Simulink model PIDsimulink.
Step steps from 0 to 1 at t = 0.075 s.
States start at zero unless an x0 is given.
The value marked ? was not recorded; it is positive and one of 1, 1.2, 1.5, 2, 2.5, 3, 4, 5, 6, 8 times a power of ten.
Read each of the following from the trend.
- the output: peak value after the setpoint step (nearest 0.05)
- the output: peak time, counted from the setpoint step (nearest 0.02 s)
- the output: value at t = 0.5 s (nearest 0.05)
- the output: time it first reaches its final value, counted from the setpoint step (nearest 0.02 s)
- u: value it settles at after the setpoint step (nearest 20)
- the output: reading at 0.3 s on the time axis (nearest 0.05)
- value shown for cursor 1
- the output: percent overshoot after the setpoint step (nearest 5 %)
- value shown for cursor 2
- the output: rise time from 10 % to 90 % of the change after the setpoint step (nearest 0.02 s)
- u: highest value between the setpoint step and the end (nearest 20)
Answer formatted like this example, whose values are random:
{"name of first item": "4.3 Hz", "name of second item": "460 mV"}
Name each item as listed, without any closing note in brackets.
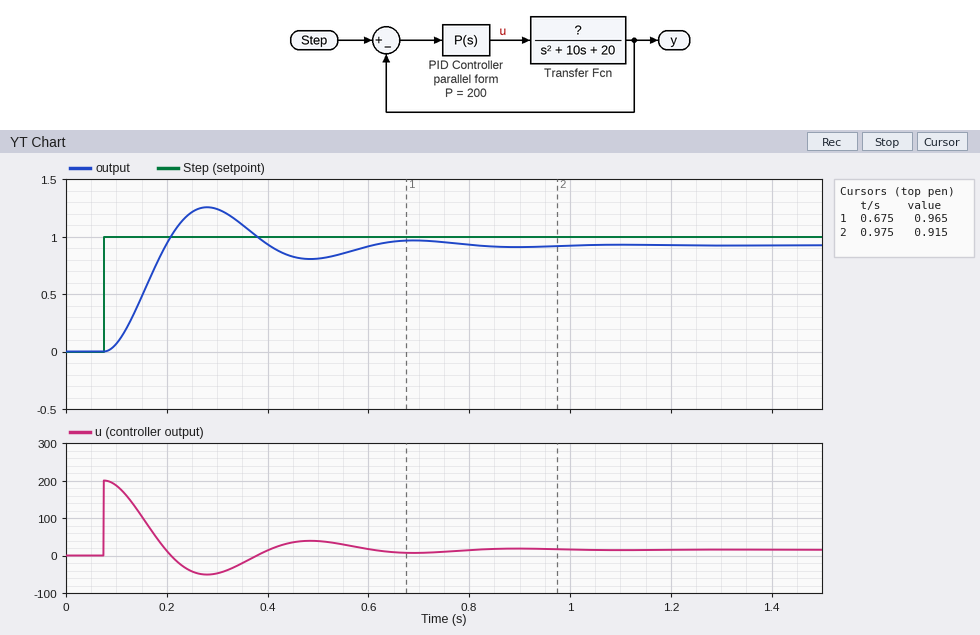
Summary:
{"the output: peak value after the setpoint step": "1.25", "the output: peak time, counted from the setpoint step": "0.20 s", "the output: value at t = 0.5 s": "0.80", "the output: time it first reaches its final value, counted from the setpoint step": "0.12 s", "u: value it settles at after the setpoint step": "20", "the output: reading at 0.3 s on the time axis": "1.25", "value shown for cursor 1": "0.965", "the output: percent overshoot after the setpoint step": "35 %", "value shown for cursor 2": "0.915", "the output: rise time from 10 % to 90 % of the change after the setpoint step": "0.08 s", "u: highest value between the setpoint step and the end": "200"}
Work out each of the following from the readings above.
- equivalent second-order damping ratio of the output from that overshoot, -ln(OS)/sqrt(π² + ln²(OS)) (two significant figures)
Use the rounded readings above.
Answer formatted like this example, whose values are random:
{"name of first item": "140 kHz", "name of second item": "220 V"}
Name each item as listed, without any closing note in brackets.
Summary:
{"equivalent second-order damping ratio of the output from that overshoot, -ln(OS)/sqrt(π² + ln²(OS))": "0.32"}
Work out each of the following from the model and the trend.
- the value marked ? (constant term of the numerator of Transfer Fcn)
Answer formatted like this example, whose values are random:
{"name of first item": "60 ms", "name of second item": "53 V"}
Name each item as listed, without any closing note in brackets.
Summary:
{"the value marked ?": "1.2"}
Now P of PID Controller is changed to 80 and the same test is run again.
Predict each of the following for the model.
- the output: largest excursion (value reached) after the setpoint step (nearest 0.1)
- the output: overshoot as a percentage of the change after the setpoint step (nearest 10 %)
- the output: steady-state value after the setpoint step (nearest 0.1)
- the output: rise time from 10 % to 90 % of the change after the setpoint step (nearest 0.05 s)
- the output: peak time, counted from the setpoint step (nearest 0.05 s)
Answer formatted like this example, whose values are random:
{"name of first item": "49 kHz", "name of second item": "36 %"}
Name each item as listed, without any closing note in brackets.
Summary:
{"the output: largest excursion (value reached) after the setpoint step": "1.0", "the output: overshoot as a percentage of the change after the setpoint step": "20 %", "the output: steady-state value after the setpoint step": "0.8", "the output: rise time from 10 % to 90 % of the change after the setpoint step": "0.15 s", "the output: peak time, counted from the setpoint step": "0.35 s"}
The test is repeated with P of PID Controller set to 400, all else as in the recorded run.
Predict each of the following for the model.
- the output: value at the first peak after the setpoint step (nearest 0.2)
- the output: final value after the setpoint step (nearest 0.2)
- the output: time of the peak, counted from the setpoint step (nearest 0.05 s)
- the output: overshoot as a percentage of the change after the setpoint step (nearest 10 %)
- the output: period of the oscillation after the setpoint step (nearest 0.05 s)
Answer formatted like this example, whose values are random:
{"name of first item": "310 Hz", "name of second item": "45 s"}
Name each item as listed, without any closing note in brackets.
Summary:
{"the output: value at the first peak after the setpoint step": "1.4", "the output: final value after the setpoint step": "1.0", "the output: time of the peak, counted from the setpoint step": "0.15 s", "the output: overshoot as a percentage of the change after the setpoint step": "50 %", "the output: period of the oscillation after the setpoint step": "0.30 s"}
